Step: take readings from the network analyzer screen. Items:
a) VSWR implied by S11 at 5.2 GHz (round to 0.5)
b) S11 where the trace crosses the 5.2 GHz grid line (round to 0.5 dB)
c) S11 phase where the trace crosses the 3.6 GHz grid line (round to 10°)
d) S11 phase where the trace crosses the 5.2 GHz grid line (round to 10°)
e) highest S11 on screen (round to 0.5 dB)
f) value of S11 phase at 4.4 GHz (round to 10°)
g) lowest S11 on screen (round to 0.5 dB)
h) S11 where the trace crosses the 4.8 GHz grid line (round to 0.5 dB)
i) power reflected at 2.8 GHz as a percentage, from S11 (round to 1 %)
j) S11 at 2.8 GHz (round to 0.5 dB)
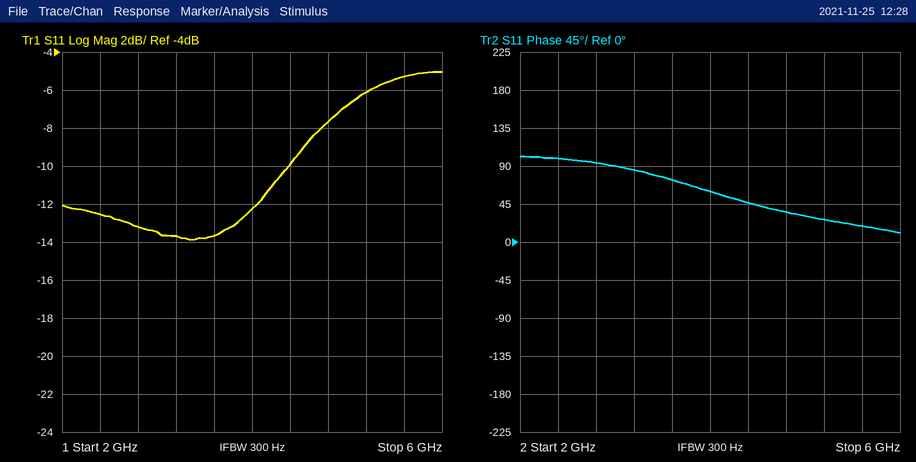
3.0
-6.0 dB
70°
30°
-5.0 dB
50°
-14.0 dB
-7.5 dB
5 %
-13.0 dB
